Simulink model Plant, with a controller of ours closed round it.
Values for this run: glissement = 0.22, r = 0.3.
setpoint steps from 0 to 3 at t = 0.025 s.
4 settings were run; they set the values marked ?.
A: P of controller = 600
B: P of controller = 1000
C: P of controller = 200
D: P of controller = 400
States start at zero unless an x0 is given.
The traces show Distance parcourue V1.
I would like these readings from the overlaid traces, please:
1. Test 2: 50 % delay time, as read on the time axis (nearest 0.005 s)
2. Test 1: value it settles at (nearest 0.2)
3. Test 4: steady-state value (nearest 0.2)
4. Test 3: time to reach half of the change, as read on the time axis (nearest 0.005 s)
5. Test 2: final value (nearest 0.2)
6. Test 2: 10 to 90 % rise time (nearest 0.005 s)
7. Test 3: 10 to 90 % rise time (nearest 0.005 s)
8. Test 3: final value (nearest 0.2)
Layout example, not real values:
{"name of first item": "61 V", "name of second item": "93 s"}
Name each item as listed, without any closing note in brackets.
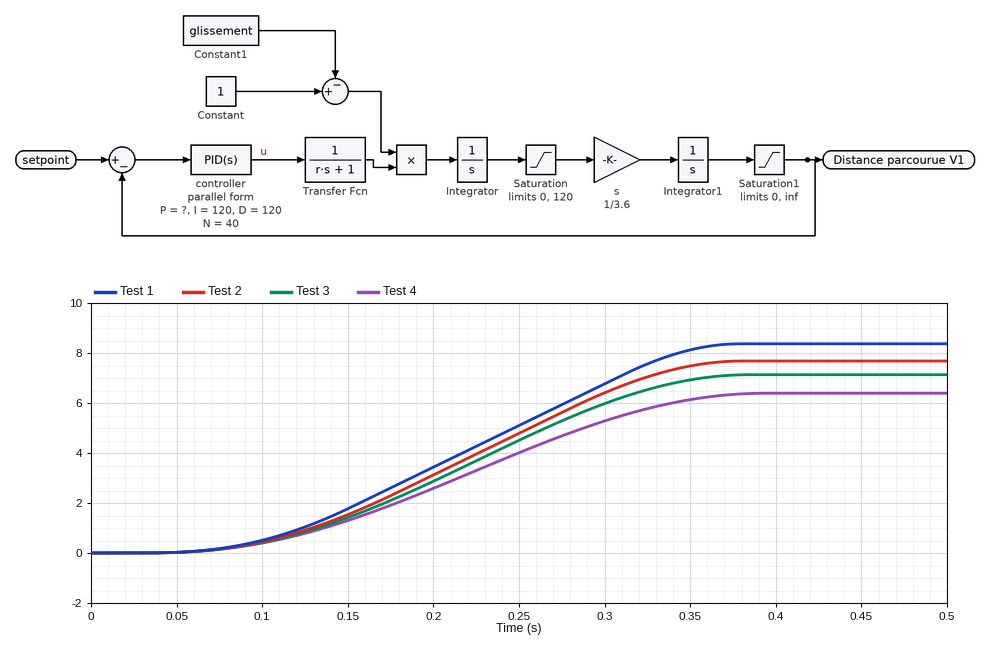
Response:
{"Test 2: 50 % delay time, as read on the time axis": "0.220 s", "Test 1: value it settles at": "8.4", "Test 4: steady-state value": "6.4", "Test 3: time to reach half of the change, as read on the time axis": "0.220 s", "Test 2: final value": "7.6", "Test 2: 10 to 90 % rise time": "0.200 s", "Test 3: 10 to 90 % rise time": "0.200 s", "Test 3: final value": "7.2"}
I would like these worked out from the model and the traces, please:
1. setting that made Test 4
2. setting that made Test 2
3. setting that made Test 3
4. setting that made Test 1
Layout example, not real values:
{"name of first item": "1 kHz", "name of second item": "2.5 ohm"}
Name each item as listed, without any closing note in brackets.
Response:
{"setting that made Test 4": "C", "setting that made Test 2": "A", "setting that made Test 3": "D", "setting that made Test 1": "B"}
